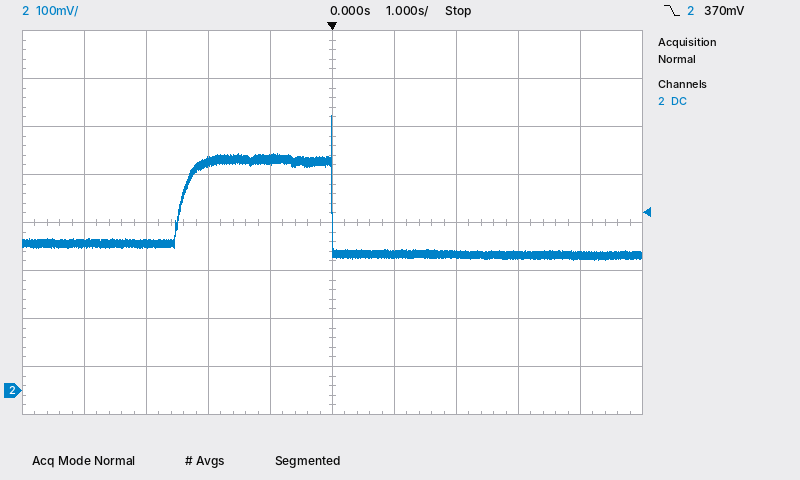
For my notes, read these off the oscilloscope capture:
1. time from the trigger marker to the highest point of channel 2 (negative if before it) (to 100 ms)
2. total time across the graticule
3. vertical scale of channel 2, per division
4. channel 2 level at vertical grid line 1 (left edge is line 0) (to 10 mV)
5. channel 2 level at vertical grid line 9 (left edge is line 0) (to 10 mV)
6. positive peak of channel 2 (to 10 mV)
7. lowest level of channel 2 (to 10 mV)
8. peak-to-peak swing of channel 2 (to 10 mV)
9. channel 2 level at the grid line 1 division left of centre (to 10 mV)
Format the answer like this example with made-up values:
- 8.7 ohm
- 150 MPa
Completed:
- 0.0 s
- 10 s
- 100 mV
- 310 mV
- 280 mV
- 570 mV
- 270 mV
- 300 mV
- 480 mV
